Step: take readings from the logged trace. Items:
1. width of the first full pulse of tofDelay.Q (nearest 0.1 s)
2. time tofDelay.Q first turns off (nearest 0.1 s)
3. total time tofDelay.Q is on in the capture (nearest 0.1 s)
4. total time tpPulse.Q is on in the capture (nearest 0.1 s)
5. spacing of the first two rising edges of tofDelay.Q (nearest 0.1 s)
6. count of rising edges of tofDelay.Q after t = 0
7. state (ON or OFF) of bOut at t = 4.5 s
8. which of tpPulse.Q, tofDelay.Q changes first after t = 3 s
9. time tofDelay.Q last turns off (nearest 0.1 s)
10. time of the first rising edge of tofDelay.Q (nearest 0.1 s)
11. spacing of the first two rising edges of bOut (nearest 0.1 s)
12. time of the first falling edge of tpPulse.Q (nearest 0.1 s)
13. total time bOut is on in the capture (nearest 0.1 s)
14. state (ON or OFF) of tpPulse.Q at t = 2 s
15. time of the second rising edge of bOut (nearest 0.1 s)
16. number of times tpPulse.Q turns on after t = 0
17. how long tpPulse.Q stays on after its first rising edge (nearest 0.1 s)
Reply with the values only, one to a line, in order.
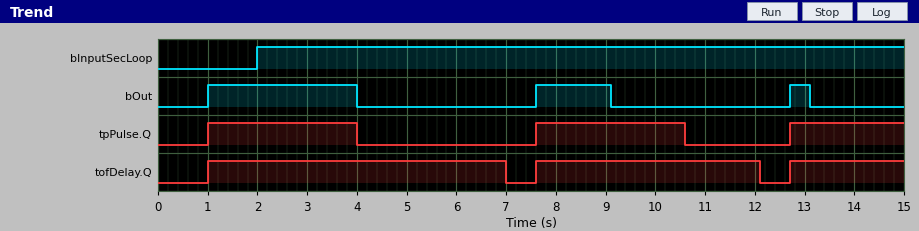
6.0 s
7.0 s
12.8 s
8.3 s
6.6 s
3
OFF
tpPulse.Q
12.1 s
1.0 s
6.6 s
4.0 s
4.9 s
ON
7.6 s
3
3.0 s
